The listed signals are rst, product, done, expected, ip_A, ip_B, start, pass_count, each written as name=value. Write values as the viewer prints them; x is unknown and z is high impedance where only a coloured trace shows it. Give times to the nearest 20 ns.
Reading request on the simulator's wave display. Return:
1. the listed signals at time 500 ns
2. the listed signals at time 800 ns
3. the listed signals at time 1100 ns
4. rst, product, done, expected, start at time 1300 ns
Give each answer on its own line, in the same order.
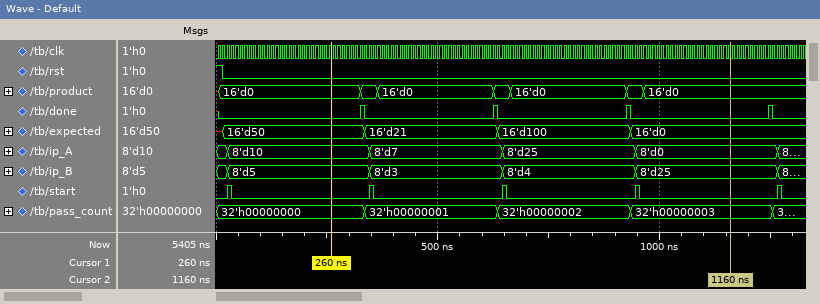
rst=0, product=16'd0, done=0, expected=16'd21, ip_A=8'd7, ip_B=8'd3, start=0, pass_count=32'h00000001
rst=0, product=16'd0, done=0, expected=16'd100, ip_A=8'd25, ip_B=8'd4, start=0, pass_count=32'h00000002
rst=0, product=16'd0, done=0, expected=16'd0, ip_A=8'd0, ip_B=8'd25, start=0, pass_count=32'h00000003
rst=0, product=16'd0, done=0, expected=16'd0, start=0
